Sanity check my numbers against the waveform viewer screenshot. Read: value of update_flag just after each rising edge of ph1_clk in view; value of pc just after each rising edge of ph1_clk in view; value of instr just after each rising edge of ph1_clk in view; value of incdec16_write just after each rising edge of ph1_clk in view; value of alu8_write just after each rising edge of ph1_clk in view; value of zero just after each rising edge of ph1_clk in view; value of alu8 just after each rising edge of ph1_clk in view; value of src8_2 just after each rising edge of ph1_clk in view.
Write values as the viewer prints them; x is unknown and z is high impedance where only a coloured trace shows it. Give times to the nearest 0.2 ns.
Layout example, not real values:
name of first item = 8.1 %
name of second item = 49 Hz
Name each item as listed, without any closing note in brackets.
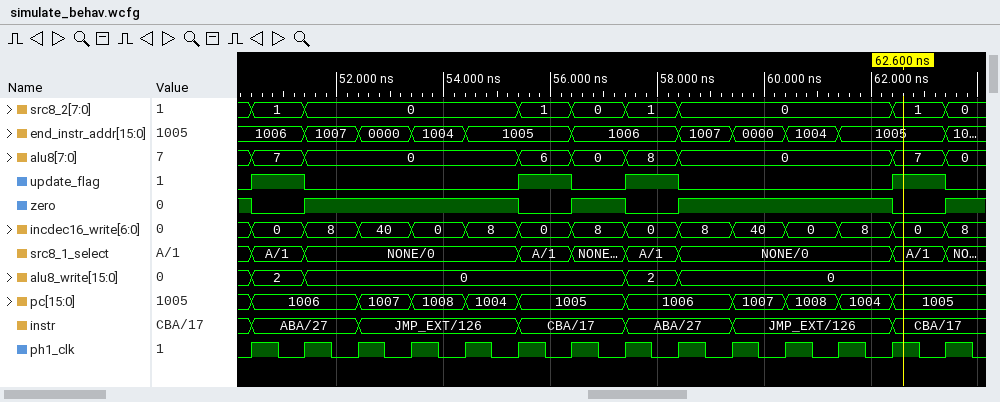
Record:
value of update_flag just after each rising edge of ph1_clk in view = 1 0 0 0 0 1 0 1 0 0 0 0 1 0
value of pc just after each rising edge of ph1_clk in view = 1006, 1006, 1007, 1008, 1004, 1005, 1005, 1006, 1006, 1007, 1008, 1004, 1005, 1005
value of instr just after each rising edge of ph1_clk in view = ABA/27, ABA/27, JMP_EXT/126, JMP_EXT/126, JMP_EXT/126, CBA/17, CBA/17, ABA/27, ABA/27, JMP_EXT/126, JMP_EXT/126, JMP_EXT/126, CBA/17, CBA/17
value of incdec16_write just after each rising edge of ph1_clk in view = 0, 8, 40, 0, 8, 0, 8, 0, 8, 40, 0, 8, 0, 8
value of alu8_write just after each rising edge of ph1_clk in view = 2, 0, 0, 0, 0, 0, 0, 2, 0, 0, 0, 0, 0, 0
value of zero just after each rising edge of ph1_clk in view = 0 1 1 1 1 0 1 0 1 1 1 1 0 1
value of alu8 just after each rising edge of ph1_clk in view = 7, 0, 0, 0, 0, 6, 0, 8, 0, 0, 0, 0, 7, 0
value of src8_2 just after each rising edge of ph1_clk in view = 1, 0, 0, 0, 0, 1, 0, 1, 0, 0, 0, 0, 1, 0
